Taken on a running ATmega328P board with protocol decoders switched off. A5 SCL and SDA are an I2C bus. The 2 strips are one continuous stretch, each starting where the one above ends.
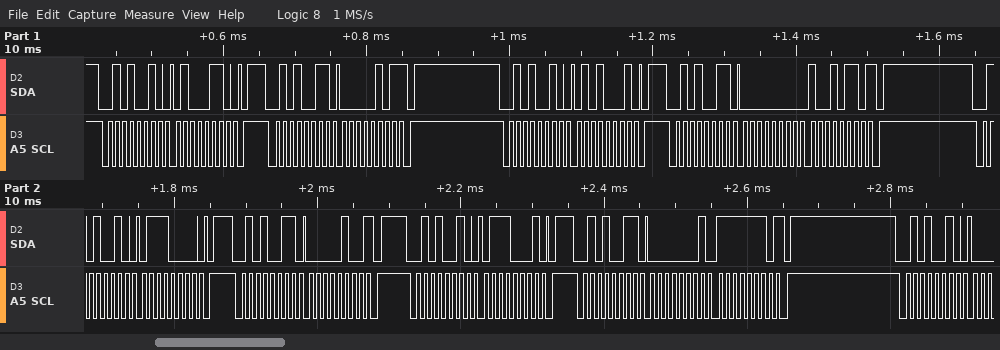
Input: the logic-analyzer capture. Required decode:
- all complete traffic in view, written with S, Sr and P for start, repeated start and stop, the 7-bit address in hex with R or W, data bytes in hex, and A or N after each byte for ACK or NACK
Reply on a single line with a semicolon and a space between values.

S 29W A 46 A P S 29R A 05 N P S 29W A 51 A P S 29R A 00 A 96 N P S 29W A 70 A P S 29R A 04 N P S 29W A 71 A P S 29R A 01 A FE N P S 29W A
